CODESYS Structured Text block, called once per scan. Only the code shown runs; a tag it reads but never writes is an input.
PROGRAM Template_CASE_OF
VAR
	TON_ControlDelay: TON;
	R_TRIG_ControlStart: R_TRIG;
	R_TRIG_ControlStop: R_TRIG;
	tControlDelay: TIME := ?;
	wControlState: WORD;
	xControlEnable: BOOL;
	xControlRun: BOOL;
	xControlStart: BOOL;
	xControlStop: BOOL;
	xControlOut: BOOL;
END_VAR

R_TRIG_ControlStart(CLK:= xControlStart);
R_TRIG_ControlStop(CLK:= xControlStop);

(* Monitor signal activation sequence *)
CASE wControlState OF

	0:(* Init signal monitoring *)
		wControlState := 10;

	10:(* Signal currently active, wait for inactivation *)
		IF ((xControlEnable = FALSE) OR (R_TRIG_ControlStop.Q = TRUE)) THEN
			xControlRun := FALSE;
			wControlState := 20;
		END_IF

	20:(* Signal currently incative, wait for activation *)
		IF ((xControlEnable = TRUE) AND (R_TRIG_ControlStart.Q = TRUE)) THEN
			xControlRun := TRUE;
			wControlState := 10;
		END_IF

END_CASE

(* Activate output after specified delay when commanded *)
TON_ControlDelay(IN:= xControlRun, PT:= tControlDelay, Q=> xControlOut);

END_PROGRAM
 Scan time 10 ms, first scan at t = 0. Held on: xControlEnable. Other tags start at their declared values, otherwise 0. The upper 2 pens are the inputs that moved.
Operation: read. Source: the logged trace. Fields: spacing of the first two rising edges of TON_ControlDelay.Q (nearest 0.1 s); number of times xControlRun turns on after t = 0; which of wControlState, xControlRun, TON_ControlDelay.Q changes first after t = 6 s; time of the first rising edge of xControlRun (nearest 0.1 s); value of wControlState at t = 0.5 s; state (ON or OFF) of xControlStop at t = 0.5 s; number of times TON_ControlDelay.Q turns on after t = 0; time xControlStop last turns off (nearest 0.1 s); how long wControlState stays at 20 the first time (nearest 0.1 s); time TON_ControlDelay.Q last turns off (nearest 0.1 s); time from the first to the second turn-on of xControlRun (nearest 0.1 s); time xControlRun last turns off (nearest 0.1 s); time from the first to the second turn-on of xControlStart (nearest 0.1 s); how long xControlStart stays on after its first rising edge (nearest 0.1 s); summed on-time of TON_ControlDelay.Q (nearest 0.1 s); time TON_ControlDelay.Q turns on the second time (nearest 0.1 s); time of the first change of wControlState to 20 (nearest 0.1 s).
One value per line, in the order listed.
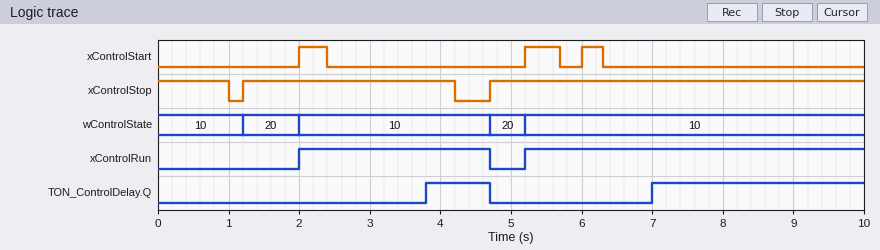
3.2 s
2
TON_ControlDelay.Q
2.0 s
10
ON
2
4.2 s
0.8 s
4.7 s
3.2 s
4.7 s
3.2 s
0.4 s
3.9 s
7.0 s
1.2 s
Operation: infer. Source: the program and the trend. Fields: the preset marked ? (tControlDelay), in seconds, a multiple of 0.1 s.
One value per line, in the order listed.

1.8 s
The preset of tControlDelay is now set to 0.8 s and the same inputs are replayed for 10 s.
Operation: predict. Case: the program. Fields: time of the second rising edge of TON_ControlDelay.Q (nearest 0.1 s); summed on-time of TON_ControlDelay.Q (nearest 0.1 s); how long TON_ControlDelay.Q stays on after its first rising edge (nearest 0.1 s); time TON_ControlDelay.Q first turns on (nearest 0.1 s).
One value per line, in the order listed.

6.0 s
5.9 s
1.9 s
2.8 s
